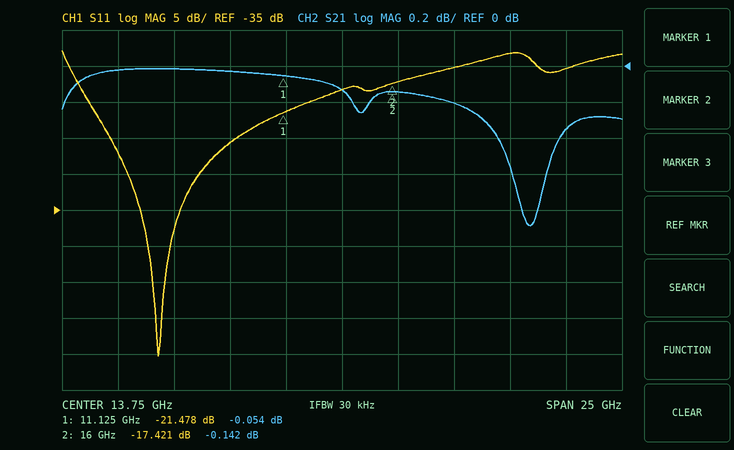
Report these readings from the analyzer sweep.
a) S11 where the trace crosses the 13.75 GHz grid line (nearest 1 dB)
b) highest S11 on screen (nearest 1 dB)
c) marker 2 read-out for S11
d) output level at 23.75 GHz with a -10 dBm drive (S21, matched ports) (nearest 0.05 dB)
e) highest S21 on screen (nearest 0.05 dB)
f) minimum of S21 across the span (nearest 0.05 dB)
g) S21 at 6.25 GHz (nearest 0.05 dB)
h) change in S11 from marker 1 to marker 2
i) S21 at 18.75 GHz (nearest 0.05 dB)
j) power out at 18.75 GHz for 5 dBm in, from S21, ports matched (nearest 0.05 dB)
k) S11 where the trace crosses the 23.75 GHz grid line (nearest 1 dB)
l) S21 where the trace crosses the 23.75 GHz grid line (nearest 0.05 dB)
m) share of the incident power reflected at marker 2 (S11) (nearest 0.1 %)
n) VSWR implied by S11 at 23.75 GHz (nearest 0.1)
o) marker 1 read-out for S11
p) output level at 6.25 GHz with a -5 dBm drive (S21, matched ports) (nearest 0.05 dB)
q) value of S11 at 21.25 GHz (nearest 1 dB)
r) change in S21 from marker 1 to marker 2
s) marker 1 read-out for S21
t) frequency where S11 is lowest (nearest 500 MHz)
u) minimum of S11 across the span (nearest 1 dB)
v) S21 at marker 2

-18 dB
-13 dB
-17.421 dB
-10.35 dBm
0.00 dB
-0.90 dB
0.00 dB
4.057 dB
-0.20 dB
4.80 dBm
-15 dB
-0.35 dB
1.8 %
1.4
-21.478 dB
-5.00 dBm
-13 dB
-0.088 dB
-0.054 dB
5.5 GHz
-55 dB
-0.142 dB
